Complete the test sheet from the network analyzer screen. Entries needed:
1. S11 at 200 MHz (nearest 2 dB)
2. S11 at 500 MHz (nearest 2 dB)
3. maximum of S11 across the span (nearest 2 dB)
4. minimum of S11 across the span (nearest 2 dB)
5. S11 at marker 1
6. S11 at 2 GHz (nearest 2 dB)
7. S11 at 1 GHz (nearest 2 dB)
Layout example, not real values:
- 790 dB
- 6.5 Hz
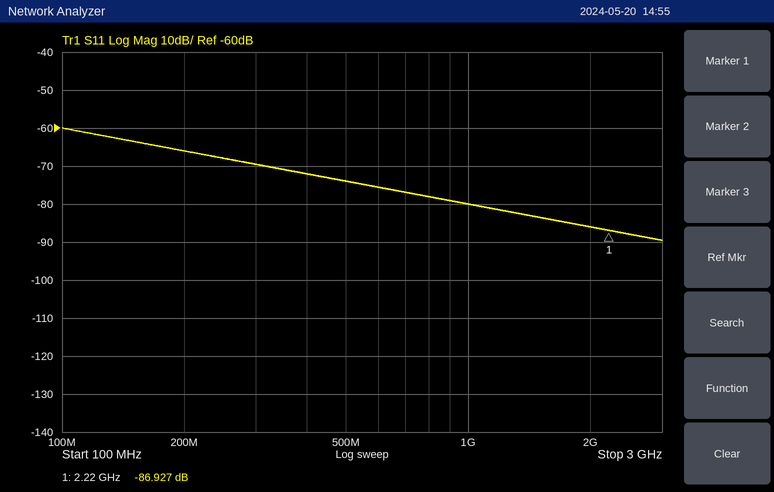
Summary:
- -66 dB
- -74 dB
- -60 dB
- -90 dB
- -86.927 dB
- -86 dB
- -80 dB
